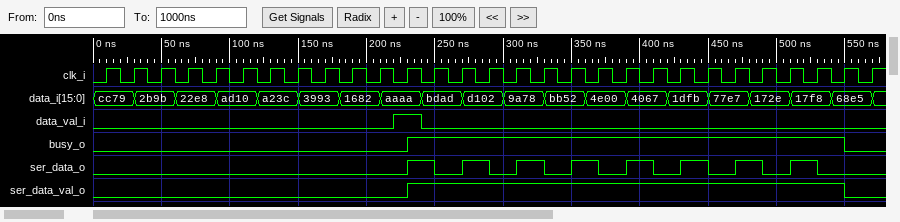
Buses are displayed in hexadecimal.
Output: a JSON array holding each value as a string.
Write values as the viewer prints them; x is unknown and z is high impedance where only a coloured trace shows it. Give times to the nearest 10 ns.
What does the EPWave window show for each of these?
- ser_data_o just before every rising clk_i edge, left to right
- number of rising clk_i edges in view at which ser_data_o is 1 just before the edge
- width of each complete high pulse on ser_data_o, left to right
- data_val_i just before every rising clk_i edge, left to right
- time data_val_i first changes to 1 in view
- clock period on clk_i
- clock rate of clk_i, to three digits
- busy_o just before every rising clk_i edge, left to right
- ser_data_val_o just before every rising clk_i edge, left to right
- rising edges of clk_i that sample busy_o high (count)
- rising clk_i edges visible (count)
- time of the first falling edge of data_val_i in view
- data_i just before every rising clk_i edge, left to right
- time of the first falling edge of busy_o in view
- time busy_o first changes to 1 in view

["0 0 0 0 0 0 0 0 0 0 0 0 1 0 1 0 1 0 1 0 1 0 1 0 1 0 1 0 0", "8", "20 ns, 20 ns, 20 ns, 20 ns, 20 ns, 20 ns, 20 ns, 20 ns", "0 0 0 0 0 0 0 0 0 0 0 1 0 0 0 0 0 0 0 0 0 0 0 0 0 0 0 0 0", "220 ns", "20 ns", "50.0 MHz", "0 0 0 0 0 0 0 0 0 0 0 0 1 1 1 1 1 1 1 1 1 1 1 1 1 1 1 1 0", "0 0 0 0 0 0 0 0 0 0 0 0 1 1 1 1 1 1 1 1 1 1 1 1 1 1 1 1 0", "16", "29", "240 ns", "cc79, cc79, 2b9b, 22e8, 22e8, ad10, a23c, a23c, 3993, 1682, 1682, aaaa, bdad, bdad, d102, 9a78, 9a78, bb52, 4e00, 4e00, 4067, 1dfb, 1dfb, 77e7, 172e, 172e, 17f8, 68e5, 68e5", "550 ns", "230 ns"]
